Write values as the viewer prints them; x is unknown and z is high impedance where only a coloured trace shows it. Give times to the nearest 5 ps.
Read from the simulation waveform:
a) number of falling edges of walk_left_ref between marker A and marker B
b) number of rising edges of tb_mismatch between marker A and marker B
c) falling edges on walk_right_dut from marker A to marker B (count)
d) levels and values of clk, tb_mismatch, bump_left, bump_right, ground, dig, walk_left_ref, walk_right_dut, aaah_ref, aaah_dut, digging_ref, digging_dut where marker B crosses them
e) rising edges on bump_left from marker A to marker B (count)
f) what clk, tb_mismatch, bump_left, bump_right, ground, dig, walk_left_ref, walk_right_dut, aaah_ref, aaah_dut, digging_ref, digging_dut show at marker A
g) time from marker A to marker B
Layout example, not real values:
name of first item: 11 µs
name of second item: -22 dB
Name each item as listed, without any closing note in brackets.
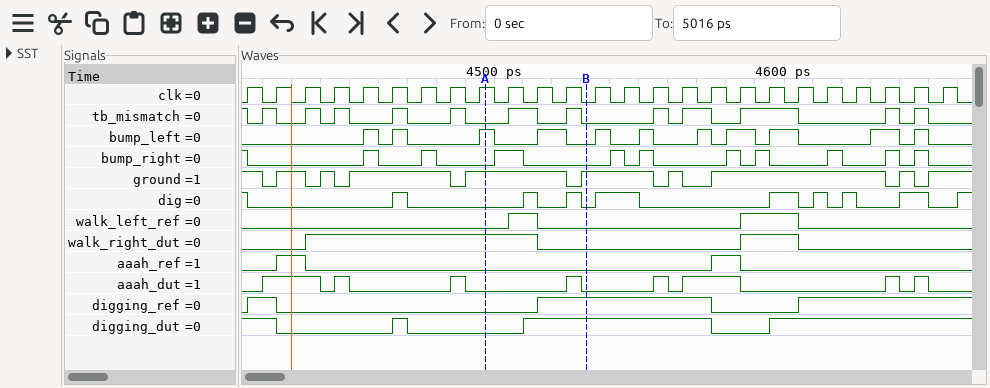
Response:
number of falling edges of walk_left_ref between marker A and marker B: 1
number of rising edges of tb_mismatch between marker A and marker B: 2
falling edges on walk_right_dut from marker A to marker B: 1
levels and values of clk, tb_mismatch, bump_left, bump_right, ground, dig, walk_left_ref, walk_right_dut, aaah_ref, aaah_dut, digging_ref, digging_dut where marker B crosses them: clk=0, tb_mismatch=0, bump_left=0, bump_right=0, ground=1, dig=0, walk_left_ref=0, walk_right_dut=0, aaah_ref=0, aaah_dut=0, digging_ref=1, digging_dut=1
rising edges on bump_left from marker A to marker B: 1
what clk, tb_mismatch, bump_left, bump_right, ground, dig, walk_left_ref, walk_right_dut, aaah_ref, aaah_dut, digging_ref, digging_dut show at marker A: clk=1, tb_mismatch=0, bump_left=1, bump_right=0, ground=1, dig=0, walk_left_ref=0, walk_right_dut=1, aaah_ref=0, aaah_dut=0, digging_ref=0, digging_dut=0
time from marker A to marker B: 35 ps
